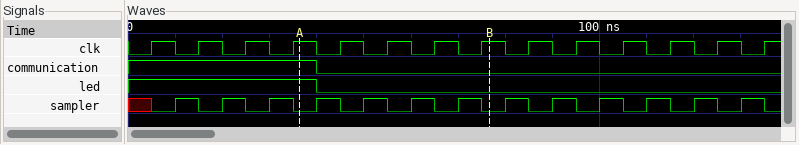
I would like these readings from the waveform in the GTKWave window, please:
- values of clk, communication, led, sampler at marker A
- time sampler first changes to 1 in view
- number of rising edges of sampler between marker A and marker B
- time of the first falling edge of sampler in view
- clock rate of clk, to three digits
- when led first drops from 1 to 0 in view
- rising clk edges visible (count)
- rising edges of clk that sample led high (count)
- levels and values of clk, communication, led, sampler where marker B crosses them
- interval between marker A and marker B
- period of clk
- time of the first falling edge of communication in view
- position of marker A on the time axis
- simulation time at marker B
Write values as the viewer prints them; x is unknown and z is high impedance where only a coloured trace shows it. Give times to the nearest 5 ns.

clk=1, communication=1, led=1, sampler=0
10 ns
4
15 ns
100 MHz
40 ns
14
4
clk=1, communication=0, led=0, sampler=0
40 ns
10 ns
40 ns
35 ns
75 ns
